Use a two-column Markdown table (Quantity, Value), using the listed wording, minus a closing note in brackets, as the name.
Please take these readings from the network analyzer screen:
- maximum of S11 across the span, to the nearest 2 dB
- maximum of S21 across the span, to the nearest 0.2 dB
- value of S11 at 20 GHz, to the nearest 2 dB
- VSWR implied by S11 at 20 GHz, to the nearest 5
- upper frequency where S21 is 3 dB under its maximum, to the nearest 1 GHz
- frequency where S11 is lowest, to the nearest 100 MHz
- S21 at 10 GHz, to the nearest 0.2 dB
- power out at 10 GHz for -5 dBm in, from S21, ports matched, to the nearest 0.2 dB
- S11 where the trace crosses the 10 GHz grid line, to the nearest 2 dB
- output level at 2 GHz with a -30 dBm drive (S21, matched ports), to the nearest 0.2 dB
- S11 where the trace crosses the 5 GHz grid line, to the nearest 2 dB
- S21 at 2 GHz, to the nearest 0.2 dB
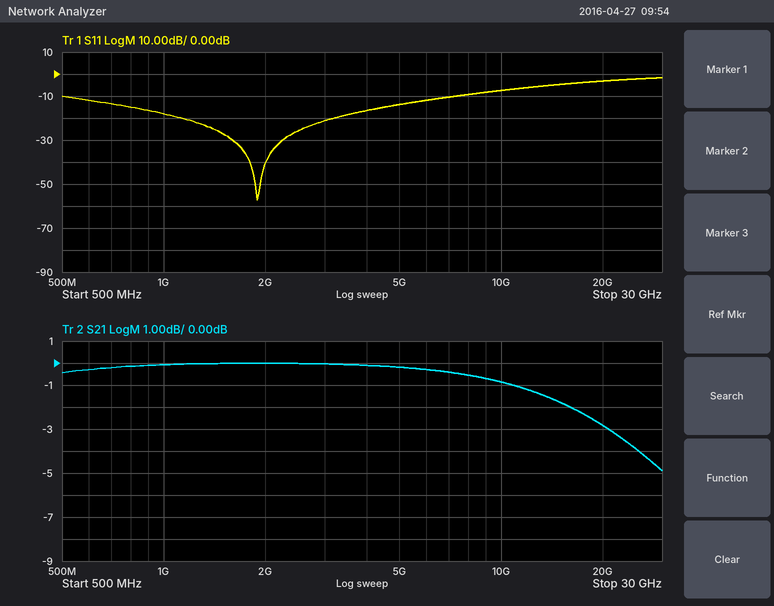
| Quantity | Value |
|---|---|
| maximum of S11 across the span, to the nearest 2 dB | -2 dB |
| maximum of S21 across the span, to the nearest 0.2 dB | 0.0 dB |
| value of S11 at 20 GHz, to the nearest 2 dB | -4 dB |
| VSWR implied by S11 at 20 GHz, to the nearest 5 | 5 |
| upper frequency where S21 is 3 dB under its maximum, to the nearest 1 GHz | 21 GHz |
| frequency where S11 is lowest, to the nearest 100 MHz | 1.9 GHz |
| S21 at 10 GHz, to the nearest 0.2 dB | -0.8 dB |
| power out at 10 GHz for -5 dBm in, from S21, ports matched, to the nearest 0.2 dB | -5.8 dBm |
| S11 where the trace crosses the 10 GHz grid line, to the nearest 2 dB | -8 dB |
| output level at 2 GHz with a -30 dBm drive (S21, matched ports), to the nearest 0.2 dB | -30.0 dBm |
| S11 where the trace crosses the 5 GHz grid line, to the nearest 2 dB | -14 dB |
| S21 at 2 GHz, to the nearest 0.2 dB | 0.0 dB |
